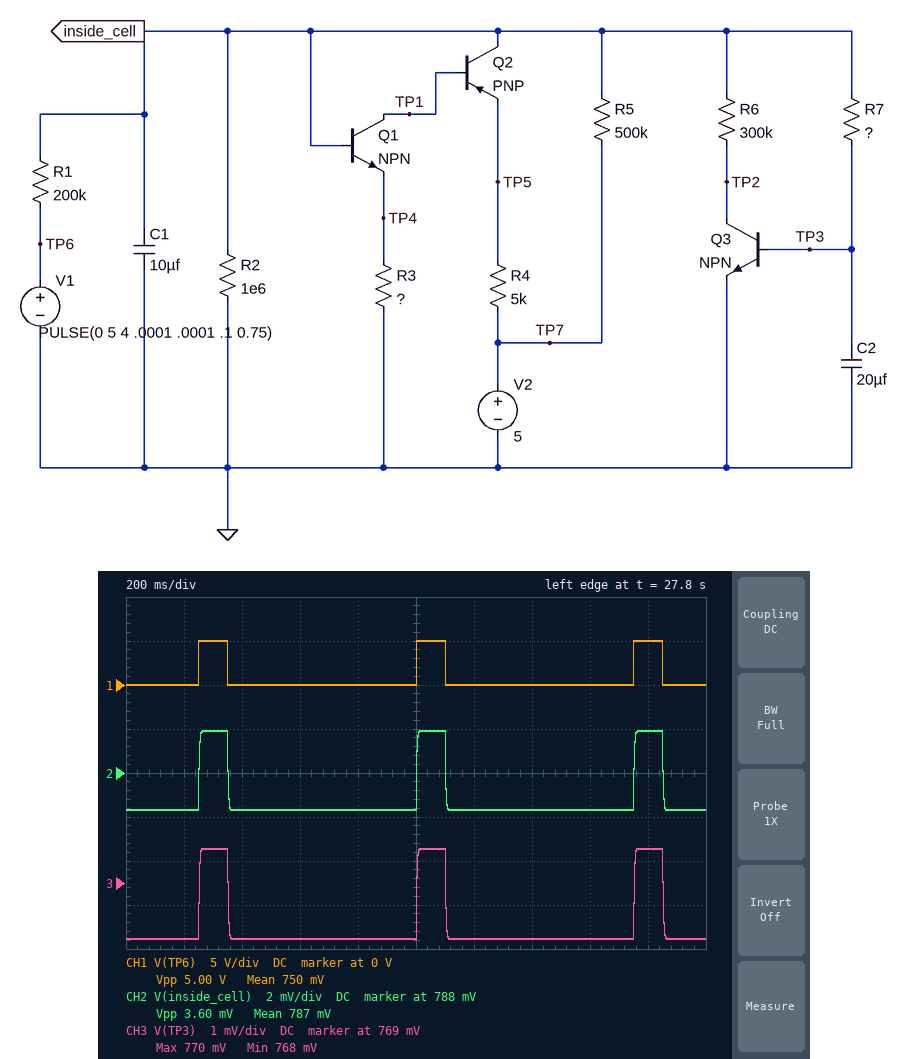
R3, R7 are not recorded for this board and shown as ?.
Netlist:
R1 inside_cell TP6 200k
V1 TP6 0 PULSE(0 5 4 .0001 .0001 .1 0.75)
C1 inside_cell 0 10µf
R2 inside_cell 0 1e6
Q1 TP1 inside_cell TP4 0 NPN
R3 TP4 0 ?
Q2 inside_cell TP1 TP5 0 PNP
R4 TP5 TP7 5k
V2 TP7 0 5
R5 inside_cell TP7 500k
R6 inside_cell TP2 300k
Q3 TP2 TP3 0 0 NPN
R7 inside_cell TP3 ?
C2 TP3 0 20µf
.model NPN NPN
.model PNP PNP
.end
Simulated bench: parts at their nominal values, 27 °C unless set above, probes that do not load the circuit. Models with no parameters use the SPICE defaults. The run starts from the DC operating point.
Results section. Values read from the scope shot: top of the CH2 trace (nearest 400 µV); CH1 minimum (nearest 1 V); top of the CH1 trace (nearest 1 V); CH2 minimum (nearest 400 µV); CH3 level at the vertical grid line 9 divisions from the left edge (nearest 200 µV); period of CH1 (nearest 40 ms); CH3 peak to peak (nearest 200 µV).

790.0 mV
0 V
5 V
786.4 mV
769.8 mV
760 ms
2.0 mV
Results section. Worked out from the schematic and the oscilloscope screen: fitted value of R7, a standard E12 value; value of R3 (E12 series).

47 Ω
39 kΩ
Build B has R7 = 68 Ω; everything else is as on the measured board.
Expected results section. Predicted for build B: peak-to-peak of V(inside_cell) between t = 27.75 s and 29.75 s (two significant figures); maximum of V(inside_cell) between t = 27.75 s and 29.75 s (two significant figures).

4.4 mV
800 mV
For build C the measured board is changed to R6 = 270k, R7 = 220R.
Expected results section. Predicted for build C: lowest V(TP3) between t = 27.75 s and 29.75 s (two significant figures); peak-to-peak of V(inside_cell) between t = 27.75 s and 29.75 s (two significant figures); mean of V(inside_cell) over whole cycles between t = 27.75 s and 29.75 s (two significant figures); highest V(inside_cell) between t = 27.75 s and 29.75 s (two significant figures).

780 mV
6.9 mV
950 mV
960 mV
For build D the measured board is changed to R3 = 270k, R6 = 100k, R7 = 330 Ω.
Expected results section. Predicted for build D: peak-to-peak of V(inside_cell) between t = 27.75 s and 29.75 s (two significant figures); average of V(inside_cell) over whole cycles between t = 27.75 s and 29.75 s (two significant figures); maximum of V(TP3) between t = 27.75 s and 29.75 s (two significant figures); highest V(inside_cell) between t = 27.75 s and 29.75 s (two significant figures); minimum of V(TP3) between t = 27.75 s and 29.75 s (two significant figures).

22 mV
740 mV
730 mV
760 mV
720 mV
